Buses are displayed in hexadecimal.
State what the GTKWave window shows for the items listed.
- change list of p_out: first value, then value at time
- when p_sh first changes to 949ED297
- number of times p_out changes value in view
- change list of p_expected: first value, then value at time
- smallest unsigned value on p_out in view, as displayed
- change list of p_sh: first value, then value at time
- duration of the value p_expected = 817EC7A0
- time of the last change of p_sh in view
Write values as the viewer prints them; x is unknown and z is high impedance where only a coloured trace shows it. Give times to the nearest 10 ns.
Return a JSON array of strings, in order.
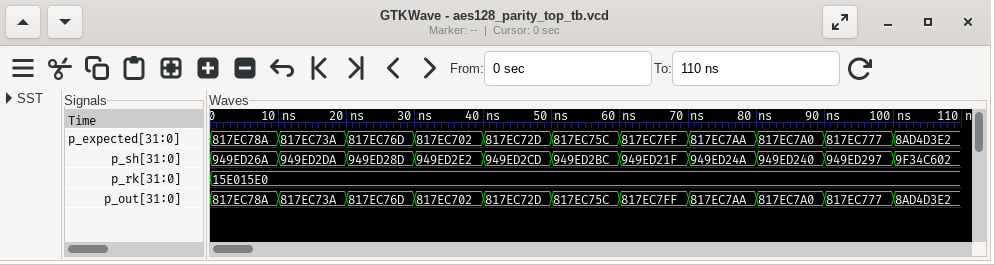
["817EC78A, 817EC73A at 10 ns, 817EC76D at 20 ns, 817EC702 at 30 ns, 817EC72D at 40 ns, 817EC75C at 50 ns, 817EC7FF at 60 ns, 817EC7AA at 70 ns, 817EC7A0 at 80 ns, 817EC777 at 90 ns, 8AD4D3E2 at 100 ns", "90 ns", "10", "817EC78A, 817EC73A at 10 ns, 817EC76D at 20 ns, 817EC702 at 30 ns, 817EC72D at 40 ns, 817EC75C at 50 ns, 817EC7FF at 60 ns, 817EC7AA at 70 ns, 817EC7A0 at 80 ns, 817EC777 at 90 ns, 8AD4D3E2 at 100 ns", "817EC702", "949ED26A, 949ED2DA at 10 ns, 949ED28D at 20 ns, 949ED2E2 at 30 ns, 949ED2CD at 40 ns, 949ED2BC at 50 ns, 949ED21F at 60 ns, 949ED24A at 70 ns, 949ED240 at 80 ns, 949ED297 at 90 ns, 9F34C602 at 100 ns", "10 ns", "100 ns"]
